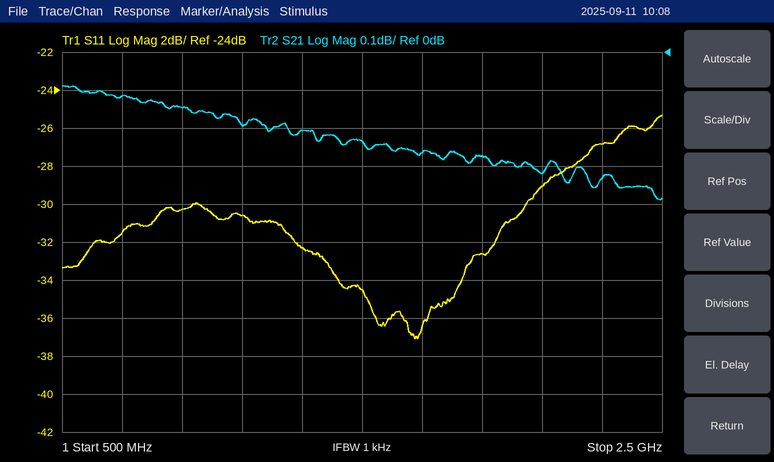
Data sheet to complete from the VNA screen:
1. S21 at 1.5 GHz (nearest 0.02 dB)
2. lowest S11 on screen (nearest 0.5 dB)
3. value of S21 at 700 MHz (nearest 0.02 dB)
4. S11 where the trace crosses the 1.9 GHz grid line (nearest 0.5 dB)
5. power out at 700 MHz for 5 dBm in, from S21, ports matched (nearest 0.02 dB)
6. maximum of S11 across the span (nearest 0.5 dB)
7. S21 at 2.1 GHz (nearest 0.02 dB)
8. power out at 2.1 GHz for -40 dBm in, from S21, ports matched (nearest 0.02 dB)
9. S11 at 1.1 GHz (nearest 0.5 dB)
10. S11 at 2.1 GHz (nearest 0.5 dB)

-0.24 dB
-37.0 dB
-0.12 dB
-32.5 dB
4.88 dBm
-25.5 dB
-0.32 dB
-40.32 dBm
-30.5 dB
-29.0 dB
